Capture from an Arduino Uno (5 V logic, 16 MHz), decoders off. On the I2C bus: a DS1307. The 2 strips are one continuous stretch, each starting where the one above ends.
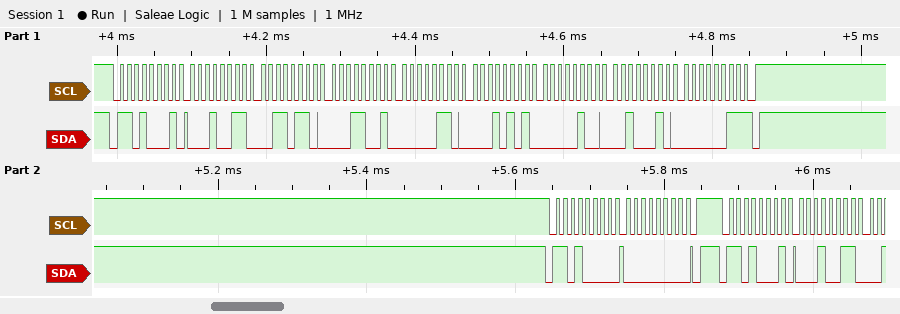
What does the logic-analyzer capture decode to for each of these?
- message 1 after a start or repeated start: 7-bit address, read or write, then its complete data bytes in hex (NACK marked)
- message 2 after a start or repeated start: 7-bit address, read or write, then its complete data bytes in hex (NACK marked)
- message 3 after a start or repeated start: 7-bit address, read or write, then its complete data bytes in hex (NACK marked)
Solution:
0x68 read: 13 36 19 06 15 04 22 03 NACK
0x68 write: 00
0x68 read: 13
